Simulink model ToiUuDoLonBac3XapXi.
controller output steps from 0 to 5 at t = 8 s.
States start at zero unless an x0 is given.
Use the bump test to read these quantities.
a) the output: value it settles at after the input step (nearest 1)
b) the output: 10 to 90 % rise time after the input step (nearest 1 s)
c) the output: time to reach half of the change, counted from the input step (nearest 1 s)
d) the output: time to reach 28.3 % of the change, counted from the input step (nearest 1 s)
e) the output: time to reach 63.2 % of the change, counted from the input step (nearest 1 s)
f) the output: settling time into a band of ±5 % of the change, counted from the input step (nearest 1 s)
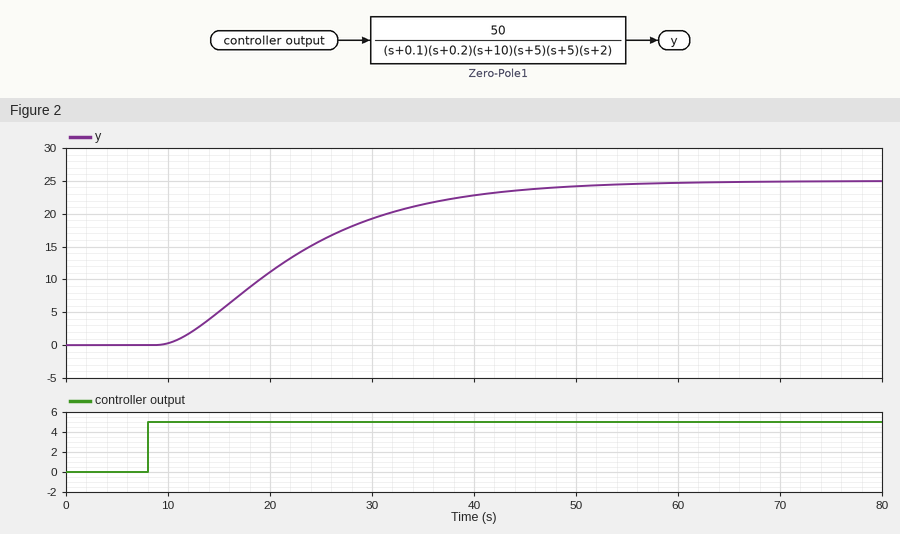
25
26 s
13 s
9 s
17 s
38 s
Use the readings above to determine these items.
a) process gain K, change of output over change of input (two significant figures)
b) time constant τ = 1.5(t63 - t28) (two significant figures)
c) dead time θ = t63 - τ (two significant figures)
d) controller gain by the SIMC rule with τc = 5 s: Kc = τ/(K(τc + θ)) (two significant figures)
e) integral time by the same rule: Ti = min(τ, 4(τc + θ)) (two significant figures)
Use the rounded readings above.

5.0
12 s
5.0 s
0.24
12 s
